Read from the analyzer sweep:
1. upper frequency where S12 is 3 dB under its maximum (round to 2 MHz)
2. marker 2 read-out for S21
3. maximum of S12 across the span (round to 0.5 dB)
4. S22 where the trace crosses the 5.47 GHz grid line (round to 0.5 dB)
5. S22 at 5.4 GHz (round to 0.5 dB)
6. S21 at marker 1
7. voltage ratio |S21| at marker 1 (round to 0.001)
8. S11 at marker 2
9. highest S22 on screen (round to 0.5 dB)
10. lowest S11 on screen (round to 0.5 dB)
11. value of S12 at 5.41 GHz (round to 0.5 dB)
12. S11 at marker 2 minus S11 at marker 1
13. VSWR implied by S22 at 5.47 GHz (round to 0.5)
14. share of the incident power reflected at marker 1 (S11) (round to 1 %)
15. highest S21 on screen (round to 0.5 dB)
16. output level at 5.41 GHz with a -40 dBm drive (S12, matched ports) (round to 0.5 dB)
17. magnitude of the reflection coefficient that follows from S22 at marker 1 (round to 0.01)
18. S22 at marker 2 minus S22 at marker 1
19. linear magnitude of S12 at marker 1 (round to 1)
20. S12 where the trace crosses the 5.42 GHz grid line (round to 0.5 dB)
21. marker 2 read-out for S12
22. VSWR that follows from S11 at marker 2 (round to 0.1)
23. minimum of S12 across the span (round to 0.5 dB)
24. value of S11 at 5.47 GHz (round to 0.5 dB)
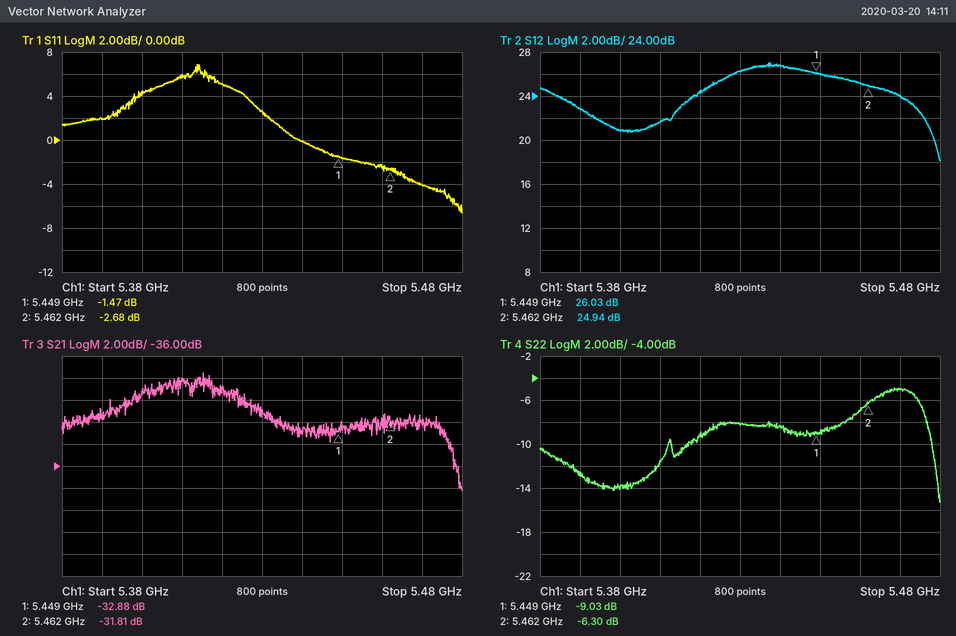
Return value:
5.470 GHz
-31.81 dB
27.0 dB
-5.0 dB
-14.0 dB
-32.88 dB
0.023
-2.68 dB
-5.0 dB
-6.5 dB
21.5 dB
-1.21 dB
3.5
71 %
-27.5 dB
-18.5 dBm
0.35
2.73 dB
20
24.5 dB
24.94 dB
6.5
18.0 dB
-4.0 dB
